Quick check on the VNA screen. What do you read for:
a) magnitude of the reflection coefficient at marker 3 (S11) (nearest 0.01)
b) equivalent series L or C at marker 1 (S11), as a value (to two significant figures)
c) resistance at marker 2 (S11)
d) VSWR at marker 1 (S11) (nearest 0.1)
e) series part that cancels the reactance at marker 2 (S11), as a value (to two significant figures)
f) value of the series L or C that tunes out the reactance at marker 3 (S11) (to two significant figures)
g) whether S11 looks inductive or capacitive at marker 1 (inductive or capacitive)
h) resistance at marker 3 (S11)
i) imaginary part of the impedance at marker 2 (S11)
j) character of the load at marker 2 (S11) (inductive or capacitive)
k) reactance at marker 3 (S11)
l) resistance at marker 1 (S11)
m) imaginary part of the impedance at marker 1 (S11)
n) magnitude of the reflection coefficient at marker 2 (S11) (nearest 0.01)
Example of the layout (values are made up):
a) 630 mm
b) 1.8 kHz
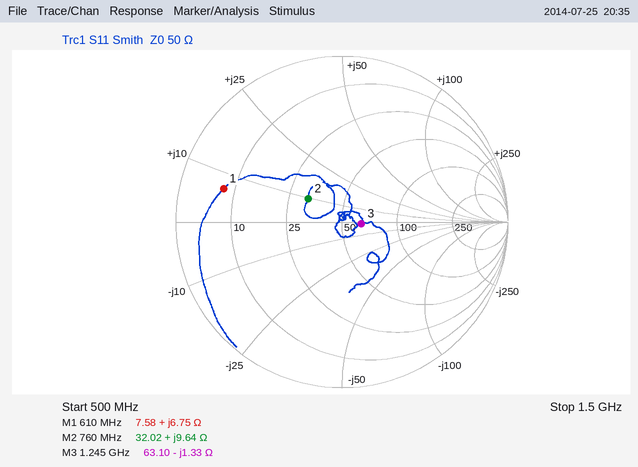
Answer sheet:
a) 0.12
b) 1.8 nH
c) 32.02 Ω
d) 6.7
e) 22 pF
f) 170 pH
g) inductive
h) 63.10 Ω
i) +9.64 Ω
j) inductive
k) -1.33 Ω
l) 7.58 Ω
m) +6.75 Ω
n) 0.25
